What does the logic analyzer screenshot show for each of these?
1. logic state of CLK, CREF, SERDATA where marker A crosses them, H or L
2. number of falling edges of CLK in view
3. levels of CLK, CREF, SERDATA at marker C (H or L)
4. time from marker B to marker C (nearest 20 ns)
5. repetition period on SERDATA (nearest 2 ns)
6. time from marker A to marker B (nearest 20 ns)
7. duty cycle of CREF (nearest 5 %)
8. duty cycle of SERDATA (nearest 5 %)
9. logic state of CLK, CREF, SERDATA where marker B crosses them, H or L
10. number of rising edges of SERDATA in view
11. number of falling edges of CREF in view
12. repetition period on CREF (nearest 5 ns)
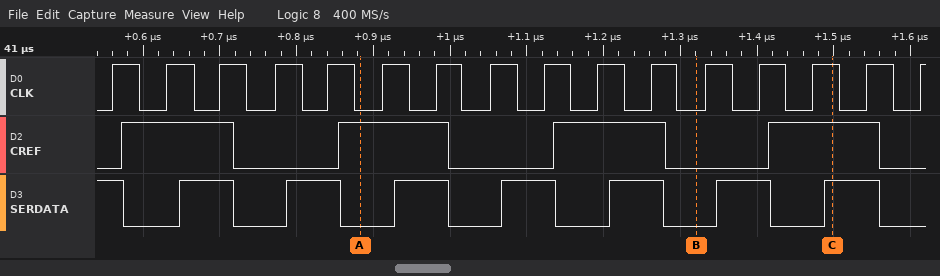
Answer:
CLK=L, CREF=H, SERDATA=L
15
CLK=H, CREF=H, SERDATA=H
180 ns
140 ns
440 ns
50 %
50 %
CLK=L, CREF=L, SERDATA=L
7
4
280 ns
